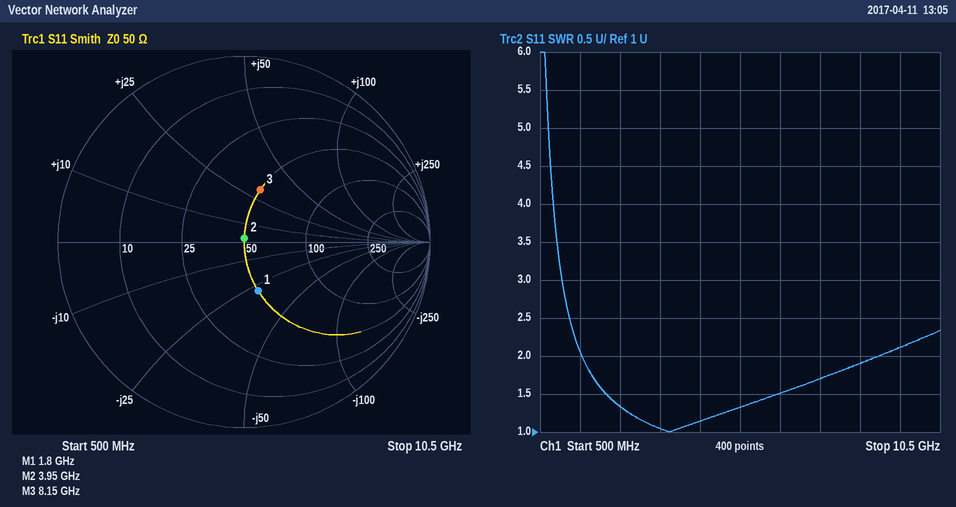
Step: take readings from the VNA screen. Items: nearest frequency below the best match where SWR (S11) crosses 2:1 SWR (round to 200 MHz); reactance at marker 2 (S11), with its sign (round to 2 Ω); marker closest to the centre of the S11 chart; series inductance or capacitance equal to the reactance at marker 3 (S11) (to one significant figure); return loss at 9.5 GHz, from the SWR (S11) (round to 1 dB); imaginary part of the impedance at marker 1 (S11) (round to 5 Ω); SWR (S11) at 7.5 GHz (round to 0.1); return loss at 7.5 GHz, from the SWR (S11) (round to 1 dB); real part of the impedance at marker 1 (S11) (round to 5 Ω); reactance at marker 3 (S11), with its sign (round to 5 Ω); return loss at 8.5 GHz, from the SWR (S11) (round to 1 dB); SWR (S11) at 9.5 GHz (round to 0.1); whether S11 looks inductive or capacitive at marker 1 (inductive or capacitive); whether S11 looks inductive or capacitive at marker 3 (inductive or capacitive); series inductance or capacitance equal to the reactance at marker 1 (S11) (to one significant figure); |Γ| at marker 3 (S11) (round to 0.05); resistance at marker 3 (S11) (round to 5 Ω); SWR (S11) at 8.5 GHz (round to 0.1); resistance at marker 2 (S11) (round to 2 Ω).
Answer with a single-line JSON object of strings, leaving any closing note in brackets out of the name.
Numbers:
{"nearest frequency below the best match where SWR (S11) crosses 2:1 SWR": "1.6 GHz", "reactance at marker 2 (S11), with its sign": "+2 Ω", "marker closest to the centre of the S11 chart": "marker 2", "series inductance or capacitance equal to the reactance at marker 3 (S11)": "600 pH", "return loss at 9.5 GHz, from the SWR (S11)": "9 dB", "imaginary part of the impedance at marker 1 (S11)": "-30 Ω", "SWR (S11) at 7.5 GHz": "1.7", "return loss at 7.5 GHz, from the SWR (S11)": "12 dB", "real part of the impedance at marker 1 (S11)": "50 Ω", "reactance at marker 3 (S11), with its sign": "+30 Ω", "return loss at 8.5 GHz, from the SWR (S11)": "10 dB", "SWR (S11) at 9.5 GHz": "2.1", "whether S11 looks inductive or capacitive at marker 1": "capacitive", "whether S11 looks inductive or capacitive at marker 3": "inductive", "series inductance or capacitance equal to the reactance at marker 1 (S11)": "3 pF", "|Γ| at marker 3 (S11)": "0.30", "resistance at marker 3 (S11)": "50 Ω", "SWR (S11) at 8.5 GHz": "1.9", "resistance at marker 2 (S11)": "50 Ω"}
